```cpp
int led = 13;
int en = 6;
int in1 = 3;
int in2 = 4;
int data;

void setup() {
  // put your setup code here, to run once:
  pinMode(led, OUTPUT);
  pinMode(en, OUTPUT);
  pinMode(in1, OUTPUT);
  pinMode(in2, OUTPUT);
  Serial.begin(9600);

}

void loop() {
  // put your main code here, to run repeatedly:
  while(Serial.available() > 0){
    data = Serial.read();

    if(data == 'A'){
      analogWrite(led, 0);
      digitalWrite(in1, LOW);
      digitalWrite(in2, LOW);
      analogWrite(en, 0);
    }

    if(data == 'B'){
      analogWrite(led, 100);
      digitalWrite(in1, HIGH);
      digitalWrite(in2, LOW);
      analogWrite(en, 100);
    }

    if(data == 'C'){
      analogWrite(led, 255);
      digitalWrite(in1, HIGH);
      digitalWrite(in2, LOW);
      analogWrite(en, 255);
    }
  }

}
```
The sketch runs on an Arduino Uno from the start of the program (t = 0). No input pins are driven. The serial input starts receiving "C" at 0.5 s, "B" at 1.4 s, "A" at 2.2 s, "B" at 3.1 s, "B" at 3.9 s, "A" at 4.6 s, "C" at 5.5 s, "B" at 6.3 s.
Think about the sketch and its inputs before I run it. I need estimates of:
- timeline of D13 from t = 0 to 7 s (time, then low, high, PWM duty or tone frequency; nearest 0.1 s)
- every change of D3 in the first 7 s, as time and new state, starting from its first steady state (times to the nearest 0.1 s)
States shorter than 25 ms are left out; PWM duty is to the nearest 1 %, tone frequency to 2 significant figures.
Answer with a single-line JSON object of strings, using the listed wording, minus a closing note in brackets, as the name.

{"timeline of D13 from t = 0 to 7 s": "0 s low; 0.5 s high; 1.4 s low; 5.5 s high; 6.3 s low", "every change of D3 in the first 7 s, as time and new state, starting from its first steady state": "0 s low; 0.5 s high; 2.2 s low; 3.1 s high; 4.6 s low; 5.5 s high"}
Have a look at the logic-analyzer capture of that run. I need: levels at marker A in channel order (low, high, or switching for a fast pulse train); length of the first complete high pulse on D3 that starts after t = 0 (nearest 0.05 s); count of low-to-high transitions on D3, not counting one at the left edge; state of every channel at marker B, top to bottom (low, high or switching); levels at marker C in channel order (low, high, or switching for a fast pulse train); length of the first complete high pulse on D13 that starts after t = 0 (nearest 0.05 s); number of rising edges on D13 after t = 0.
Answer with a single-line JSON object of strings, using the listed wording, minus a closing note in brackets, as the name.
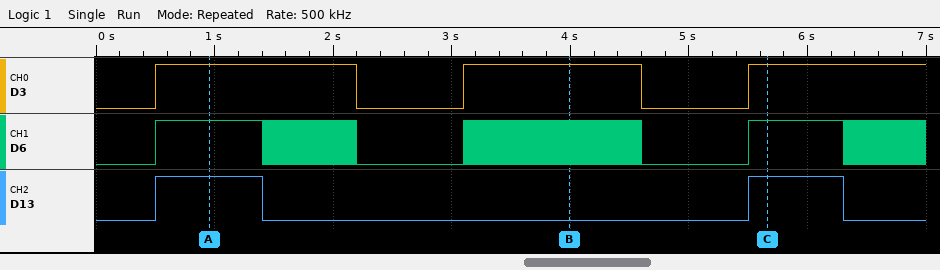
{"levels at marker A in channel order": "D3 high, D6 high, D13 high", "length of the first complete high pulse on D3 that starts after t = 0": "1.70 s", "count of low-to-high transitions on D3, not counting one at the left edge": "3", "state of every channel at marker B, top to bottom": "D3 high, D6 switching, D13 low", "levels at marker C in channel order": "D3 high, D6 high, D13 high", "length of the first complete high pulse on D13 that starts after t = 0": "0.90 s", "number of rising edges on D13 after t = 0": "2"}
